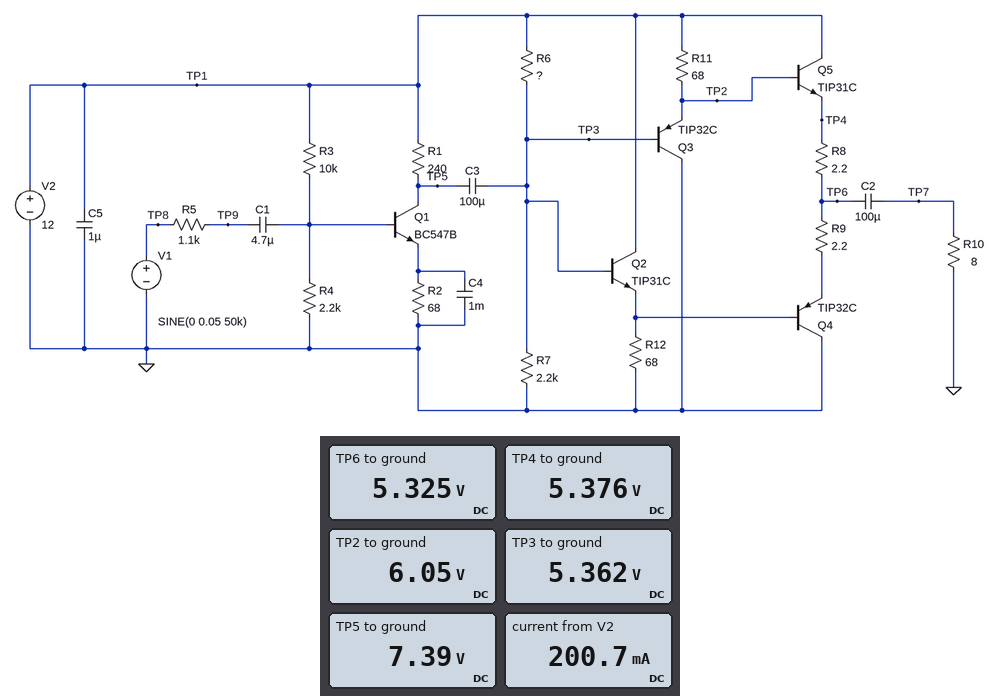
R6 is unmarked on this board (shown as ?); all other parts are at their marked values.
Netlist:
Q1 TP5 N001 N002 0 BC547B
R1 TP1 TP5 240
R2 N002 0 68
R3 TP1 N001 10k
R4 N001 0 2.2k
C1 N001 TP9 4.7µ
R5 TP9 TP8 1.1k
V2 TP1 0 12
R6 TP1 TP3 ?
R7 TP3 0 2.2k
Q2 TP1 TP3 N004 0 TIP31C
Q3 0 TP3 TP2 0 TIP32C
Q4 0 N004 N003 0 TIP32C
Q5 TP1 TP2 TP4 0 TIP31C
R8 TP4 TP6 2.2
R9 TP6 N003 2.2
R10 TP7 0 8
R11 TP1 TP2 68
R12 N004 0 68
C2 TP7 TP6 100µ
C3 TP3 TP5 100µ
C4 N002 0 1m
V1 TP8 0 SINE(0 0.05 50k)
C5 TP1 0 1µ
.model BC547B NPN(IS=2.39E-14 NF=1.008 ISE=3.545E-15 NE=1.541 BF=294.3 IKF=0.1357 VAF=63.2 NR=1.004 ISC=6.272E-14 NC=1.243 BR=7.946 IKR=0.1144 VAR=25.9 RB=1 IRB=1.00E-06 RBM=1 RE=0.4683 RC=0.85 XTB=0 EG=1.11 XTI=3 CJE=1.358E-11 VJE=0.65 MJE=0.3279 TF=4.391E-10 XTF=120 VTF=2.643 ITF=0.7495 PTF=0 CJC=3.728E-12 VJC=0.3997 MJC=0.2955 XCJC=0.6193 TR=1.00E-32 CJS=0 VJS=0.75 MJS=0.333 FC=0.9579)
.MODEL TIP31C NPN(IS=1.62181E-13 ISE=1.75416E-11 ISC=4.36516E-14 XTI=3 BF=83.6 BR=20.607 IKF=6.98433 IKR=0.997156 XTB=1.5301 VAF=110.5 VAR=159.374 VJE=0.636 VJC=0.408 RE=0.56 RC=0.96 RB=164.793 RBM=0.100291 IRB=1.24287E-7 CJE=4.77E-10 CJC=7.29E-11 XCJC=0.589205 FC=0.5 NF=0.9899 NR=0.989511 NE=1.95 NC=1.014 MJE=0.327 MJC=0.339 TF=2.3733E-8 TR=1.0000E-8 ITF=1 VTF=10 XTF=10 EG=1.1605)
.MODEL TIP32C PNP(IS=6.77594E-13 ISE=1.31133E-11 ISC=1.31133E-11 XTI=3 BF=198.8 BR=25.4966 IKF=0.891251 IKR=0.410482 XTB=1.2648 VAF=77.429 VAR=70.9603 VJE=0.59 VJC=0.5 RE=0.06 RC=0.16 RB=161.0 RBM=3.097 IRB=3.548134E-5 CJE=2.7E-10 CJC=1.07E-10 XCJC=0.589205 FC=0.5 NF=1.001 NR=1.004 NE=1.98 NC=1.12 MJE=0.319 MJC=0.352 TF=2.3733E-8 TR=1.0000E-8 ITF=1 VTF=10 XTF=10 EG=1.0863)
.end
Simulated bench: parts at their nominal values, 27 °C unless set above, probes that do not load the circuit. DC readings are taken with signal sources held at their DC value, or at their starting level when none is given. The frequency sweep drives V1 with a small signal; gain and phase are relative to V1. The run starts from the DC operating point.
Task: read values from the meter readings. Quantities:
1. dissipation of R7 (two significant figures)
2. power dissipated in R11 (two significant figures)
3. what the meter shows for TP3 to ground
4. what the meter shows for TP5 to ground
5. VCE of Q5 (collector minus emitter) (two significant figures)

13 mW
520 mW
5.362 V
7.39 V
6.6 V
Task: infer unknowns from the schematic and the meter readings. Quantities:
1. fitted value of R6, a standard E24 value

2.4 kΩ
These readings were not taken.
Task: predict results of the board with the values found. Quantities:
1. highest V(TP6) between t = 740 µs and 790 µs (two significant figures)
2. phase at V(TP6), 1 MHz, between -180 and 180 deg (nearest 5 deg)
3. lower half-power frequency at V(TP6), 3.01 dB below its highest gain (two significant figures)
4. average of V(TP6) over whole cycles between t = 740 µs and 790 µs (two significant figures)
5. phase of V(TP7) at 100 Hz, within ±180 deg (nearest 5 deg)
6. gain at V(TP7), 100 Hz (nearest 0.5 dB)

6.2 V
85 deg
40 Hz
5.3 V
-90 deg
19.0 dB
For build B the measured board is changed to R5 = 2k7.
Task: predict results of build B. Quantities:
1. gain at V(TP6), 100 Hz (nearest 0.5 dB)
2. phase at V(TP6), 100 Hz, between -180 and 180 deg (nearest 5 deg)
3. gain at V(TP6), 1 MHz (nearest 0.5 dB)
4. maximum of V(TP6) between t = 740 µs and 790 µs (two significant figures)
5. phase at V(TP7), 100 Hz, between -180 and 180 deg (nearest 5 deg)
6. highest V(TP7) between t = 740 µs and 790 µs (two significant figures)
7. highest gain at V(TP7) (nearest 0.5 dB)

20.0 dB
-165 deg
12.5 dB
5.8 V
-100 deg
440 mV
19.0 dB
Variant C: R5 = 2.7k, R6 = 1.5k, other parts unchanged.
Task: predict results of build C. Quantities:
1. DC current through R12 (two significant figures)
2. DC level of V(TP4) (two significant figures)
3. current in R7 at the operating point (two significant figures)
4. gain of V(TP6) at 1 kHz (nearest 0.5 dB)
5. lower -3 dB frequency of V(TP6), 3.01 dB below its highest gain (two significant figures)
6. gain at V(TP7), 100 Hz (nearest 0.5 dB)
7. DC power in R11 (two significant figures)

86 mA
6.6 V
3.0 mA
18.5 dB
27 Hz
12.5 dB
330 mW
